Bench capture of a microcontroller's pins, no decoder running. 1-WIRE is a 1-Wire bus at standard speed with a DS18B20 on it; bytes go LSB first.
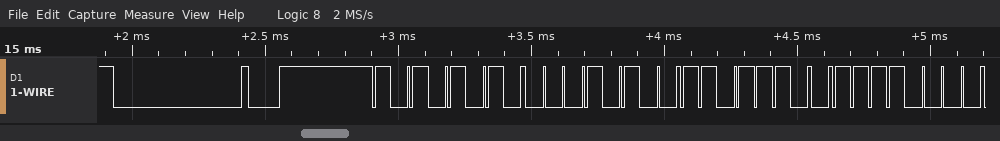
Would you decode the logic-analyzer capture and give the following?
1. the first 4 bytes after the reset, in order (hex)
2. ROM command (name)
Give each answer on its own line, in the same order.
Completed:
55 28 3B 0F
Match ROM
